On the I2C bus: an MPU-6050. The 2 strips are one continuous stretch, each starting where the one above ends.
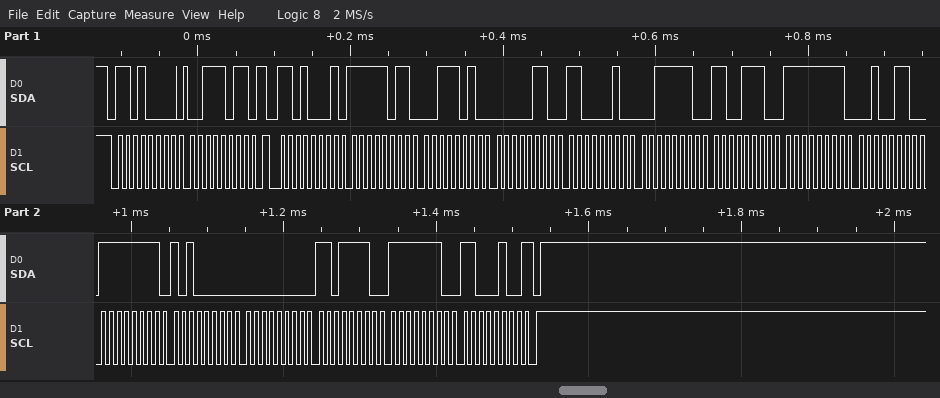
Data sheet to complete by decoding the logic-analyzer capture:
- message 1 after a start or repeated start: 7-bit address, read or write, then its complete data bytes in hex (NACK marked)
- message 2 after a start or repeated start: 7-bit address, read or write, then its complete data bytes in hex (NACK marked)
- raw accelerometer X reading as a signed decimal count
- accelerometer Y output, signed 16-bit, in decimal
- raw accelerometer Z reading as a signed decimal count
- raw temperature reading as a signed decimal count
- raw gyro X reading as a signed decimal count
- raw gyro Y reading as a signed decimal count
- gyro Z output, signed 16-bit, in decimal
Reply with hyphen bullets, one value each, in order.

- 0x68 write: 3B
- 0x68 read: FB 3A 06 C2 3E CE FF 26 FF A0 00 DE FE C4 NACK
- -1222
- 1730
- 16078
- -218
- -96
- 222
- -316
